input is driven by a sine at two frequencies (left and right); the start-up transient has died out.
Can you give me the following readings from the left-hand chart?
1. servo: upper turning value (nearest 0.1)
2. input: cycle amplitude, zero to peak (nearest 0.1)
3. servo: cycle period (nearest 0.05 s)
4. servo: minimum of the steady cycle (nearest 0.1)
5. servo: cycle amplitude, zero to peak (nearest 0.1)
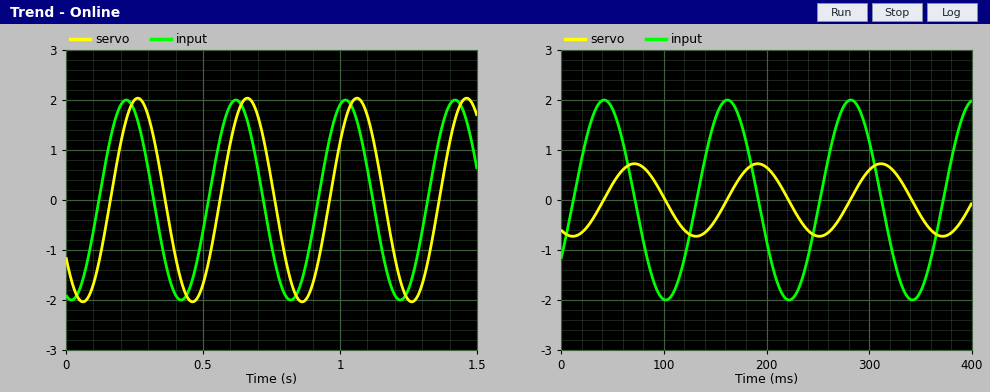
2.0
2.0
0.40 s
-2.0
2.0
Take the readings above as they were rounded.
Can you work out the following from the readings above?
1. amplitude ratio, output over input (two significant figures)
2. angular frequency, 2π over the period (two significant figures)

1.0
16 rad/s
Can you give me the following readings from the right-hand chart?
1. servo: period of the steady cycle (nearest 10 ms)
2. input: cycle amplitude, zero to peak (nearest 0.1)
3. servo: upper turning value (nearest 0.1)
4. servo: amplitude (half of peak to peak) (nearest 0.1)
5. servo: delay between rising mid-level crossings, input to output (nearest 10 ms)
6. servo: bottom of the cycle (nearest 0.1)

120 ms
2.0
0.7
0.7
30 ms
-0.7
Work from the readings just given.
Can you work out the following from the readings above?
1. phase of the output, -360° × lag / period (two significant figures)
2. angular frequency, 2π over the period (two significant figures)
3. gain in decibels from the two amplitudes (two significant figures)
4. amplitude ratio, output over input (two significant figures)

-90°
0.052 rad/ms
-9.1 dB
0.35
